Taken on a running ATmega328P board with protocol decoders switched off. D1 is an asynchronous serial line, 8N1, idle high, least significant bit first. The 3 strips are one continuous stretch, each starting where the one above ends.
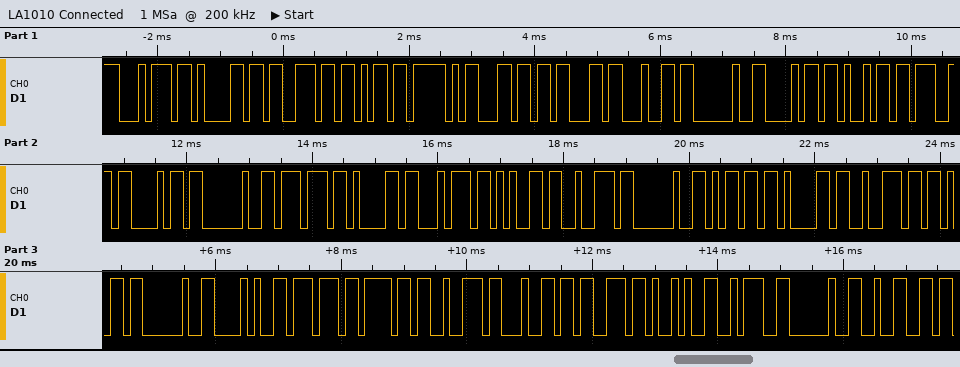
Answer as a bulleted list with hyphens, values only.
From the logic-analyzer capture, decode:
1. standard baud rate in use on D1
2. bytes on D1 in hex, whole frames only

- 9600 baud
- 74 61 73 6B 5F 6C 63 64 20 68 69 67 68 20 77 61 74 65 72 20 6D 61 72 6B 20 28 77 6F 72 64 73 29 3A 20 32
